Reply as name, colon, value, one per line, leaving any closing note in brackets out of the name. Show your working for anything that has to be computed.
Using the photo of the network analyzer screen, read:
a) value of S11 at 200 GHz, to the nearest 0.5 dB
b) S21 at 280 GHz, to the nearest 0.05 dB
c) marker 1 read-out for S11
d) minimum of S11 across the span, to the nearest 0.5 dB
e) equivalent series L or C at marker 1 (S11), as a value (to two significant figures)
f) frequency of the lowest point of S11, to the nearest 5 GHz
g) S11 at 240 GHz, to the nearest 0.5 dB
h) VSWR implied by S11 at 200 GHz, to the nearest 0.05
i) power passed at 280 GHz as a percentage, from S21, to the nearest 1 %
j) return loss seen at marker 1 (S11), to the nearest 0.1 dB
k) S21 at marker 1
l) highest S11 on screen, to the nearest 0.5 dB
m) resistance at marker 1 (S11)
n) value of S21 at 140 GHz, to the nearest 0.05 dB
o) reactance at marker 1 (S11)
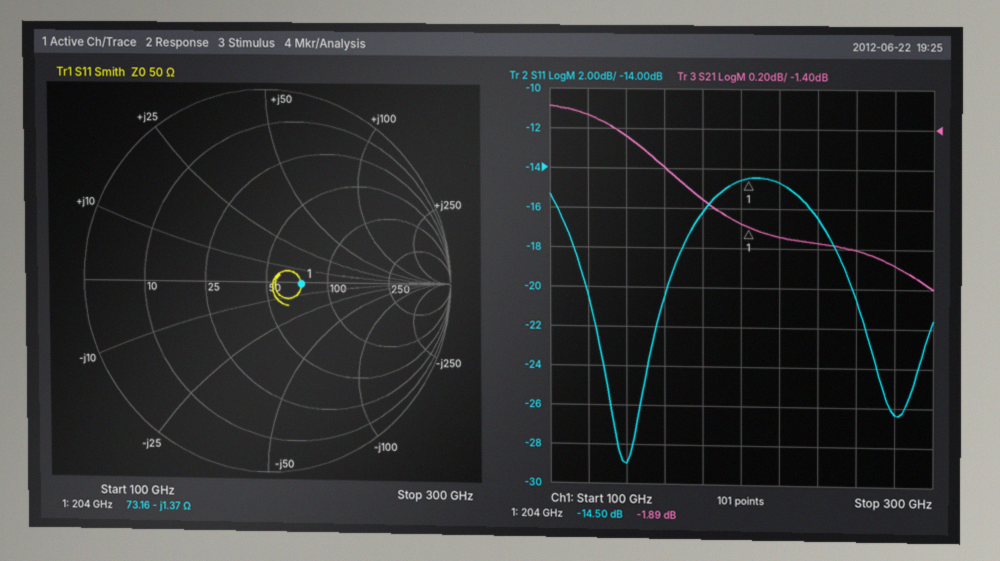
value of S11 at 200 GHz, to the nearest 0.5 dB: -14.5 dB
S21 at 280 GHz, to the nearest 0.05 dB: -2.10 dB
marker 1 read-out for S11: -14.50 dB
minimum of S11 across the span, to the nearest 0.5 dB: -29.0 dB
equivalent series L or C at marker 1 (S11), as a value: C = 1/(2π × 204 GHz × 1.37 Ω) ≈ 569 fF, so 570 fF to two significant figures
frequency of the lowest point of S11, to the nearest 5 GHz: 140 GHz
S11 at 240 GHz, to the nearest 0.5 dB: -16.5 dB
VSWR implied by S11 at 200 GHz, to the nearest 0.05: |Γ| = 10^(-14.5/20) = 0.1884; VSWR = (1 + 0.1884)/(1 − 0.1884) ≈ 1.46, so 1.45 to the nearest 0.05
power passed at 280 GHz as a percentage, from S21, to the nearest 1 %: 10^(-2.1/10) ≈ 62 %
return loss seen at marker 1 (S11), to the nearest 0.1 dB: 14.5 dB
S21 at marker 1: -1.89 dB
highest S11 on screen, to the nearest 0.5 dB: -14.5 dB
resistance at marker 1: 73.16 Ω
value of S21 at 140 GHz, to the nearest 0.05 dB: -1.45 dB
reactance at marker 1: -1.37 Ω
